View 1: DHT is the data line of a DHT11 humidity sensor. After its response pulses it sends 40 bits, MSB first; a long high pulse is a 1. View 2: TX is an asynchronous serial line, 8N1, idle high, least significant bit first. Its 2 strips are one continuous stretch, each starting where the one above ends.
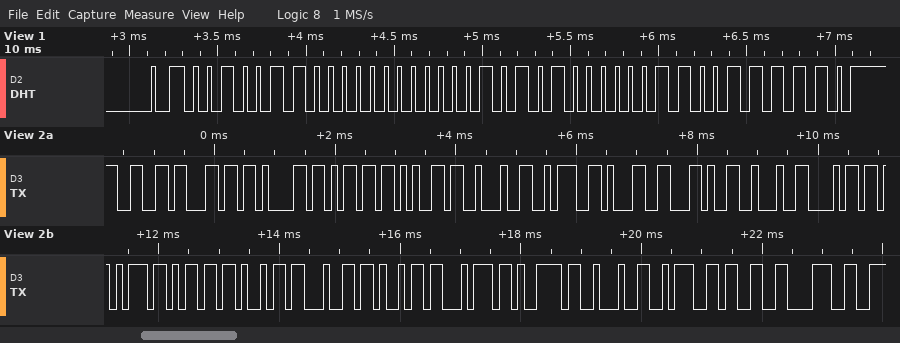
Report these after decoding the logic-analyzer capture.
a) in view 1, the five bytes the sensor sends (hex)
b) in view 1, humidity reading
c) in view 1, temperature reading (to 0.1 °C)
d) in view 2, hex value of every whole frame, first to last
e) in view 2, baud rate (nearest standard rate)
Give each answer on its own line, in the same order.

26 00 15 03 3E
38 %
21.3 °C
66 6C 61 6D 65 22 3A 31 2C 22 68 75 6D 69 64 69 74 79 22 3A 33 38
9600 baud
